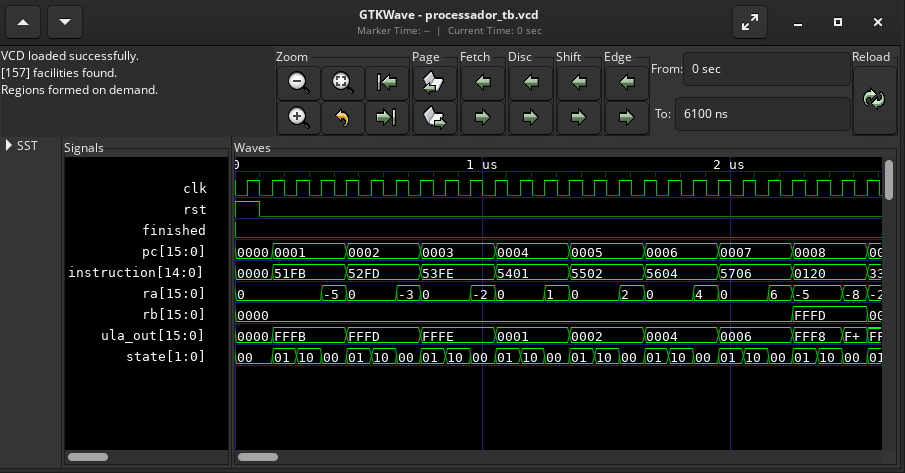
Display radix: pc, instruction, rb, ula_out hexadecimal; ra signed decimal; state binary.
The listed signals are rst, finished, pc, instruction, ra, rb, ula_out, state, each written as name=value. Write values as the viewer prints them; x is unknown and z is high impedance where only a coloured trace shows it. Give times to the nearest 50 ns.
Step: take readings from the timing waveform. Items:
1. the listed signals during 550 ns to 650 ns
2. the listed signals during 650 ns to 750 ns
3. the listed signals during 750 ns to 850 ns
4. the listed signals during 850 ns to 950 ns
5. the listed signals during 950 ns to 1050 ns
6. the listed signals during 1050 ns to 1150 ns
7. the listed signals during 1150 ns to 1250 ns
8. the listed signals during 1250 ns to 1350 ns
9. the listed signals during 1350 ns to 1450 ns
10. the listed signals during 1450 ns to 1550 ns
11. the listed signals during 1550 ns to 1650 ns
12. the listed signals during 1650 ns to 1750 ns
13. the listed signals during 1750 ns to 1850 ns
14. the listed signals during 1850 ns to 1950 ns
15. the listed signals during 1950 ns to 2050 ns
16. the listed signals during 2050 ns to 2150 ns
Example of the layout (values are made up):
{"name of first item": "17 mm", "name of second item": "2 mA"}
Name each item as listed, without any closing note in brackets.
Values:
{"the listed signals during 550 ns to 650 ns": "rst=0, finished=0, pc=0002, instruction=52FD, ra=0, rb=0000, ula_out=FFFD, state=10", "the listed signals during 650 ns to 750 ns": "rst=0, finished=0, pc=0002, instruction=52FD, ra=-3, rb=0000, ula_out=FFFD, state=00", "the listed signals during 750 ns to 850 ns": "rst=0, finished=0, pc=0003, instruction=53FE, ra=0, rb=0000, ula_out=FFFE, state=01", "the listed signals during 850 ns to 950 ns": "rst=0, finished=0, pc=0003, instruction=53FE, ra=0, rb=0000, ula_out=FFFE, state=10", "the listed signals during 950 ns to 1050 ns": "rst=0, finished=0, pc=0003, instruction=53FE, ra=-2, rb=0000, ula_out=FFFE, state=00", "the listed signals during 1050 ns to 1150 ns": "rst=0, finished=0, pc=0004, instruction=5401, ra=0, rb=0000, ula_out=0001, state=01", "the listed signals during 1150 ns to 1250 ns": "rst=0, finished=0, pc=0004, instruction=5401, ra=0, rb=0000, ula_out=0001, state=10", "the listed signals during 1250 ns to 1350 ns": "rst=0, finished=0, pc=0004, instruction=5401, ra=1, rb=0000, ula_out=0001, state=00", "the listed signals during 1350 ns to 1450 ns": "rst=0, finished=0, pc=0005, instruction=5502, ra=0, rb=0000, ula_out=0002, state=01", "the listed signals during 1450 ns to 1550 ns": "rst=0, finished=0, pc=0005, instruction=5502, ra=0, rb=0000, ula_out=0002, state=10", "the listed signals during 1550 ns to 1650 ns": "rst=0, finished=0, pc=0005, instruction=5502, ra=2, rb=0000, ula_out=0002, state=00", "the listed signals during 1650 ns to 1750 ns": "rst=0, finished=0, pc=0006, instruction=5604, ra=0, rb=0000, ula_out=0004, state=01", "the listed signals during 1750 ns to 1850 ns": "rst=0, finished=0, pc=0006, instruction=5604, ra=0, rb=0000, ula_out=0004, state=10", "the listed signals during 1850 ns to 1950 ns": "rst=0, finished=0, pc=0006, instruction=5604, ra=4, rb=0000, ula_out=0004, state=00", "the listed signals during 1950 ns to 2050 ns": "rst=0, finished=0, pc=0007, instruction=5706, ra=0, rb=0000, ula_out=0006, state=01", "the listed signals during 2050 ns to 2150 ns": "rst=0, finished=0, pc=0007, instruction=5706, ra=0, rb=0000, ula_out=0006, state=10"}
